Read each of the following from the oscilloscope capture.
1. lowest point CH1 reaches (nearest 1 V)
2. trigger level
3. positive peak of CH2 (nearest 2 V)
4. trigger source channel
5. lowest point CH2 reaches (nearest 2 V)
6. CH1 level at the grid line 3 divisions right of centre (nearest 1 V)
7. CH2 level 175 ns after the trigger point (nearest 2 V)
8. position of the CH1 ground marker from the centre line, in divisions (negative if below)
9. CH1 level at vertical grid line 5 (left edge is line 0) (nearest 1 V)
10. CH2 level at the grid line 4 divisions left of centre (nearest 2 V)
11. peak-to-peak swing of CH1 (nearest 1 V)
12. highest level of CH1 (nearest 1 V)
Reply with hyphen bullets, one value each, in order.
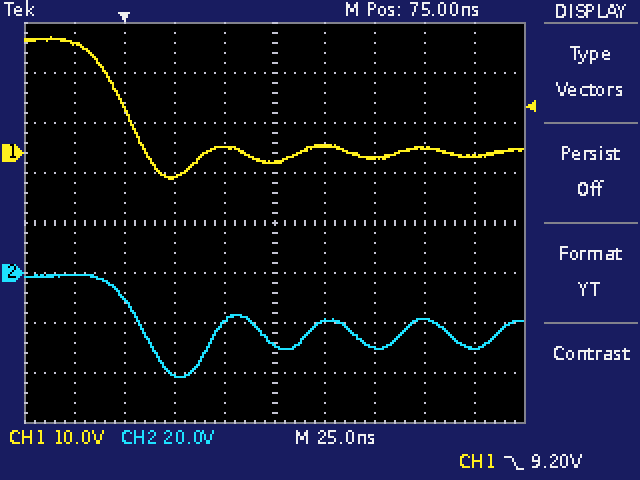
- -5 V
- 9.20 V
- 0 V
- CH1
- -42 V
- 1 V
- -30 V
- +1.4 div
- -2 V
- 0 V
- 28 V
- 23 V
